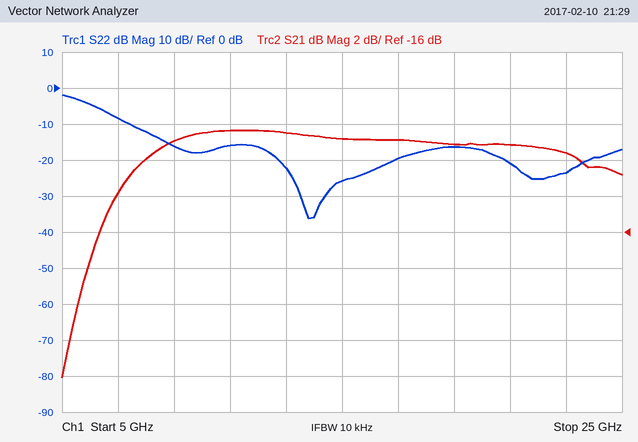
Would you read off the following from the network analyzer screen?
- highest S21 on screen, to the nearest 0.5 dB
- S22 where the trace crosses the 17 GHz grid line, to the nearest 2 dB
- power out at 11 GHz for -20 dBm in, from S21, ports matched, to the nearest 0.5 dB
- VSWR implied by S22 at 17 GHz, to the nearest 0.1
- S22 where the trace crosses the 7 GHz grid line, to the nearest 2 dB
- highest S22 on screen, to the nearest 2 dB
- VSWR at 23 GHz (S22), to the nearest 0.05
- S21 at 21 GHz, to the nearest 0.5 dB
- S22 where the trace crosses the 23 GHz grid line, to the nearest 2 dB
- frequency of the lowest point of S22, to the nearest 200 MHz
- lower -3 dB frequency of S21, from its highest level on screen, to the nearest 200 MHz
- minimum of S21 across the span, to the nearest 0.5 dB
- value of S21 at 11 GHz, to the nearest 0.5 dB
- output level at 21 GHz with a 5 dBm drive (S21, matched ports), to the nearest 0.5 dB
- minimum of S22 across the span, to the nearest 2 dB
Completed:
-10.5 dB
-20 dB
-30.5 dBm
1.2
-8 dB
-2 dB
1.15
-11.0 dB
-24 dB
13.8 GHz
7.2 GHz
-24.0 dB
-10.5 dB
-6.0 dBm
-36 dB
